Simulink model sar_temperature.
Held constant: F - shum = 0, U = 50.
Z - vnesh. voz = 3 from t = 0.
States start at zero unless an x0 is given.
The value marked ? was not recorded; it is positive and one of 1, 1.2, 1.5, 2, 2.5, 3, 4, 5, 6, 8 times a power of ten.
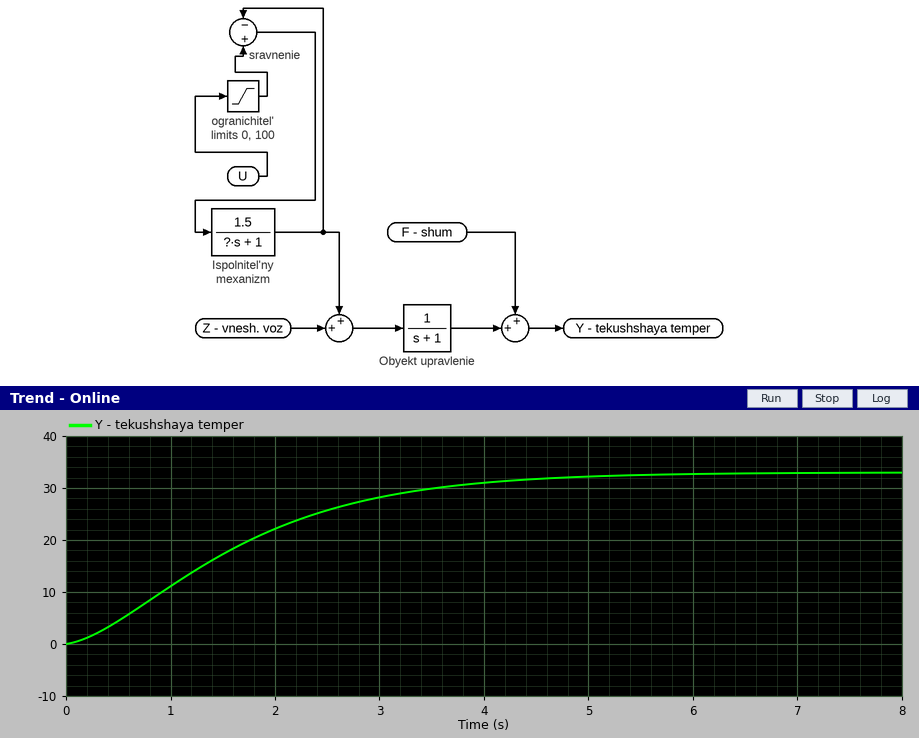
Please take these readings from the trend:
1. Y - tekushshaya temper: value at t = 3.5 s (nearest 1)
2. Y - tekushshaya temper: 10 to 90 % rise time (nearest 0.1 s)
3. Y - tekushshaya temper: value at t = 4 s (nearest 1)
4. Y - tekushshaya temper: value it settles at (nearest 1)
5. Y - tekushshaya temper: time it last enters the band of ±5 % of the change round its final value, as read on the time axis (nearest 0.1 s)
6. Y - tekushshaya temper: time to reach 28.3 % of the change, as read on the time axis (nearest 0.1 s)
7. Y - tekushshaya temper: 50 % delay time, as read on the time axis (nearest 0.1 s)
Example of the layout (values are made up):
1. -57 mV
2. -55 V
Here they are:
1. 30
2. 3.0 s
3. 31
4. 33
5. 4.2 s
6. 0.9 s
7. 1.4 s
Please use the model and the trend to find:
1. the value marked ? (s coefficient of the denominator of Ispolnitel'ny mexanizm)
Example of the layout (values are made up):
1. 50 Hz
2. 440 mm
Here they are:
1. 2
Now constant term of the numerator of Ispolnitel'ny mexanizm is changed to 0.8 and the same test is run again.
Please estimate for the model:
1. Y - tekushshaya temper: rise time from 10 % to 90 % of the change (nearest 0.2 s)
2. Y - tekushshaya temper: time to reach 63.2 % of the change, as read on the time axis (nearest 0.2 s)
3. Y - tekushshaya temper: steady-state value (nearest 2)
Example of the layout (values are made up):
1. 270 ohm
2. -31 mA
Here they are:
1. 3.6 s
2. 2.2 s
3. 26
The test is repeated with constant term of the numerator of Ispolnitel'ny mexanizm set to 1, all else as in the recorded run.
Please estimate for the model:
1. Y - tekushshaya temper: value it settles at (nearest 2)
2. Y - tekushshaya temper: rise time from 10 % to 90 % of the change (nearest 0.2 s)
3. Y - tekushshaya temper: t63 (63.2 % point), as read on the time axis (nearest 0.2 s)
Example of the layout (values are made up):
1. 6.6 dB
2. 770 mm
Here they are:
1. 28
2. 3.4 s
3. 2.0 s
